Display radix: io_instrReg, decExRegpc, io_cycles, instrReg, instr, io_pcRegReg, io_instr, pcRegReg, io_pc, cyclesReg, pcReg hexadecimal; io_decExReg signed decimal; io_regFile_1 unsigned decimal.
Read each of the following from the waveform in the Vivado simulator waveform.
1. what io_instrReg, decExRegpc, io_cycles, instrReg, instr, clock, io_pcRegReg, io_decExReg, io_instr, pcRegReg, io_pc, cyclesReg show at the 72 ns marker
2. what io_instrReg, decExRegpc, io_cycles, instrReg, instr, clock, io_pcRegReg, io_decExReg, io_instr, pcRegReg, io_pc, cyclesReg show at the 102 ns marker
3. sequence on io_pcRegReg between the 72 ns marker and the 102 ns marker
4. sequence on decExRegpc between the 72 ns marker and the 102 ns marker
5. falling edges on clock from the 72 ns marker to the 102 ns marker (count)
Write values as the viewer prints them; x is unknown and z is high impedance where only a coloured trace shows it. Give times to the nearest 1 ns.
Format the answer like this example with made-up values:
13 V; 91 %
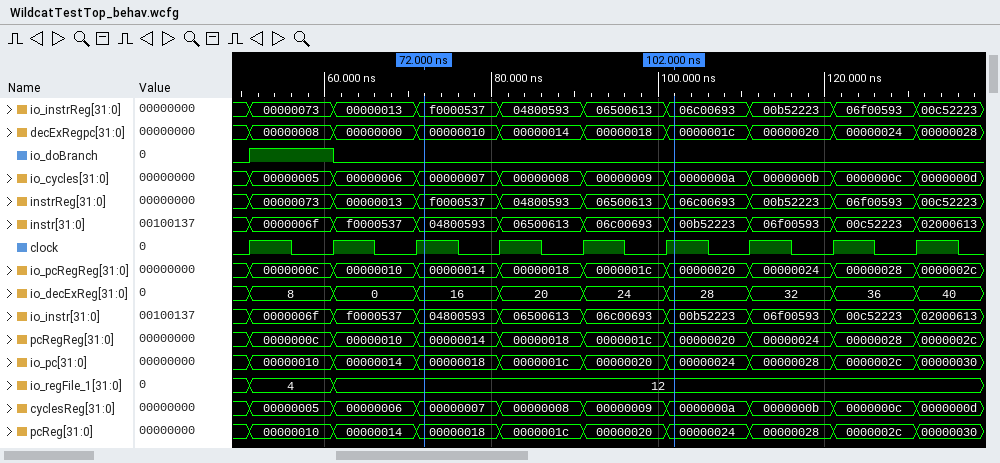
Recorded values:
io_instrReg=f0000537, decExRegpc=00000010, io_cycles=00000007, instrReg=f0000537, instr=04800593, clock=1, io_pcRegReg=00000014, io_decExReg=16, io_instr=04800593, pcRegReg=00000014, io_pc=00000018, cyclesReg=00000007; io_instrReg=06c00693, decExRegpc=0000001c, io_cycles=0000000a, instrReg=06c00693, instr=00b52223, clock=1, io_pcRegReg=00000020, io_decExReg=28, io_instr=00b52223, pcRegReg=00000020, io_pc=00000024, cyclesReg=0000000a; 00000014, 00000018, 0000001c, 00000020; 00000010, 00000014, 00000018, 0000001c; 3
